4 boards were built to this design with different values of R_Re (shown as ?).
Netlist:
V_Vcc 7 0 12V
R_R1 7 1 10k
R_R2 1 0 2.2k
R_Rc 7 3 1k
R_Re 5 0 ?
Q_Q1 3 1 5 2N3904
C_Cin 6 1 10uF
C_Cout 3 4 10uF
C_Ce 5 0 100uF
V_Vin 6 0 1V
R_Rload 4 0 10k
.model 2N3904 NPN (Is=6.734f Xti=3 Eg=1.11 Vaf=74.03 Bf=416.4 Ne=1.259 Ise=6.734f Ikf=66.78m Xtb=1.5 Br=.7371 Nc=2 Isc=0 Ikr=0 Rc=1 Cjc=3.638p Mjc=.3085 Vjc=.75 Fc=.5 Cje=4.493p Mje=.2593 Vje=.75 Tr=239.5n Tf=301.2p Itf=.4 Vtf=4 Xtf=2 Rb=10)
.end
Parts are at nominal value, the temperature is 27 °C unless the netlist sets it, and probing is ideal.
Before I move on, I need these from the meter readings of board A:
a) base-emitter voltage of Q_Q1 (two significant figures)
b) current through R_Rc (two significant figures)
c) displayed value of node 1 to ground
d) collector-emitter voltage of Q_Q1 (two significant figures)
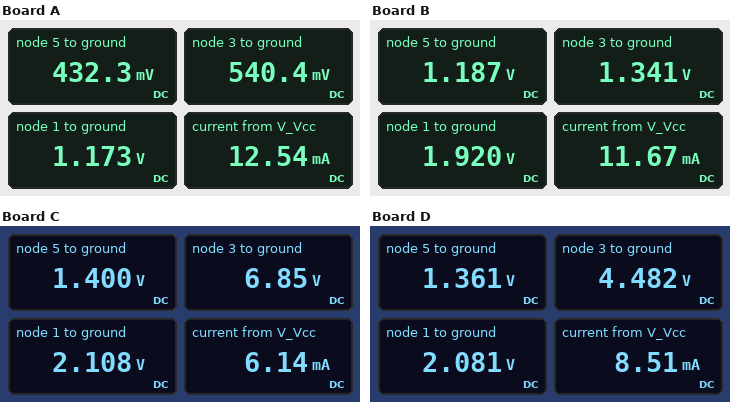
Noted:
740 mV
11 mA
1.173 V
110 mV
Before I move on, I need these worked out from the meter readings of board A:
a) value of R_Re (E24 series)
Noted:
36 Ω
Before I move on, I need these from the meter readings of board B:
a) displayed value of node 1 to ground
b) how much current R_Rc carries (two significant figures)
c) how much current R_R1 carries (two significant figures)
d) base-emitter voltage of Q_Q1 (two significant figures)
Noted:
1.920 V
11 mA
1.0 mA
730 mV
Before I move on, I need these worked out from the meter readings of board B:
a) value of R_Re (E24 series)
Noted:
110 Ω
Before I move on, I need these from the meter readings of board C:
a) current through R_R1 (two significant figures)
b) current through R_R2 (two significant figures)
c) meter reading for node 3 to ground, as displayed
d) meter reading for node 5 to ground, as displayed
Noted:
990 µA
960 µA
6.85 V
1.400 V
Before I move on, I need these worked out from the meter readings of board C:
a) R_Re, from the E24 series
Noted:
270 Ω
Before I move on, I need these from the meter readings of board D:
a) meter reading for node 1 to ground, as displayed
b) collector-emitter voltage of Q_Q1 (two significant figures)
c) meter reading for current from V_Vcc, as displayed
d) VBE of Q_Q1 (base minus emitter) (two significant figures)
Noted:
2.081 V
3.1 V
8.51 mA
720 mV
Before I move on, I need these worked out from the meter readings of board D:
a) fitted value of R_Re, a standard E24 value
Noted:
180 Ω
